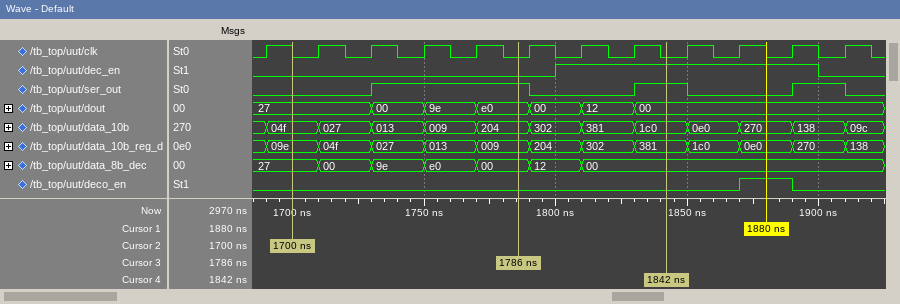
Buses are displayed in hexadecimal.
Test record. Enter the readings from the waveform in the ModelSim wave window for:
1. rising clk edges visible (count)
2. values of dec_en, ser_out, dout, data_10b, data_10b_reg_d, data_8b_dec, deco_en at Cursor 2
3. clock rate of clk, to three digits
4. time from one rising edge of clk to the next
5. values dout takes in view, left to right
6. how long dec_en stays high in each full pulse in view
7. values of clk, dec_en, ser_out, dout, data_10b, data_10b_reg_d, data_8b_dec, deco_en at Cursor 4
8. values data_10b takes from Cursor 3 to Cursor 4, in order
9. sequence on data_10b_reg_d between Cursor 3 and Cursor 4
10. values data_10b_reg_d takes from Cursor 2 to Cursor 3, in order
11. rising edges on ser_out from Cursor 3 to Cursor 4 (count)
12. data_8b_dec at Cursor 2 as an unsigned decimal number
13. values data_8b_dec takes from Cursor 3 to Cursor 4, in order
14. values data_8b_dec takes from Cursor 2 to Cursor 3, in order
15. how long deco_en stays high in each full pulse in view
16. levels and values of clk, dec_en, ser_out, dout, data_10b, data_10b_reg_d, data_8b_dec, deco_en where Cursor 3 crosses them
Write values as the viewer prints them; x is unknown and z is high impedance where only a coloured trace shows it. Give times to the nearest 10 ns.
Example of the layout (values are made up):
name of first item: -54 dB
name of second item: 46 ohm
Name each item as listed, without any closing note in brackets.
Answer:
rising clk edges visible: 12
values of dec_en, ser_out, dout, data_10b, data_10b_reg_d, data_8b_dec, deco_en at Cursor 2: dec_en=0, ser_out=0, dout=27, data_10b=04f, data_10b_reg_d=09e, data_8b_dec=27, deco_en=0
clock rate of clk, to three digits: 50.0 MHz
time from one rising edge of clk to the next: 20 ns
values dout takes in view, left to right: 27, 00, 9e, e0, 00, 12, 00
how long dec_en stays high in each full pulse in view: 100 ns
values of clk, dec_en, ser_out, dout, data_10b, data_10b_reg_d, data_8b_dec, deco_en at Cursor 4: clk=0, dec_en=1, ser_out=1, dout=00, data_10b=1c0, data_10b_reg_d=381, data_8b_dec=00, deco_en=0
values data_10b takes from Cursor 3 to Cursor 4, in order: 204, 302, 381, 1c0
sequence on data_10b_reg_d between Cursor 3 and Cursor 4: 009, 204, 302, 381
values data_10b_reg_d takes from Cursor 2 to Cursor 3, in order: 09e, 04f, 027, 013, 009
rising edges on ser_out from Cursor 3 to Cursor 4: 1
data_8b_dec at Cursor 2 as an unsigned decimal number: 39
values data_8b_dec takes from Cursor 3 to Cursor 4, in order: 00, 12, 00
values data_8b_dec takes from Cursor 2 to Cursor 3, in order: 27, 00, 9e, e0, 00
how long deco_en stays high in each full pulse in view: 20 ns
levels and values of clk, dec_en, ser_out, dout, data_10b, data_10b_reg_d, data_8b_dec, deco_en where Cursor 3 crosses them: clk=0, dec_en=0, ser_out=1, dout=e0, data_10b=204, data_10b_reg_d=009, data_8b_dec=00, deco_en=0
